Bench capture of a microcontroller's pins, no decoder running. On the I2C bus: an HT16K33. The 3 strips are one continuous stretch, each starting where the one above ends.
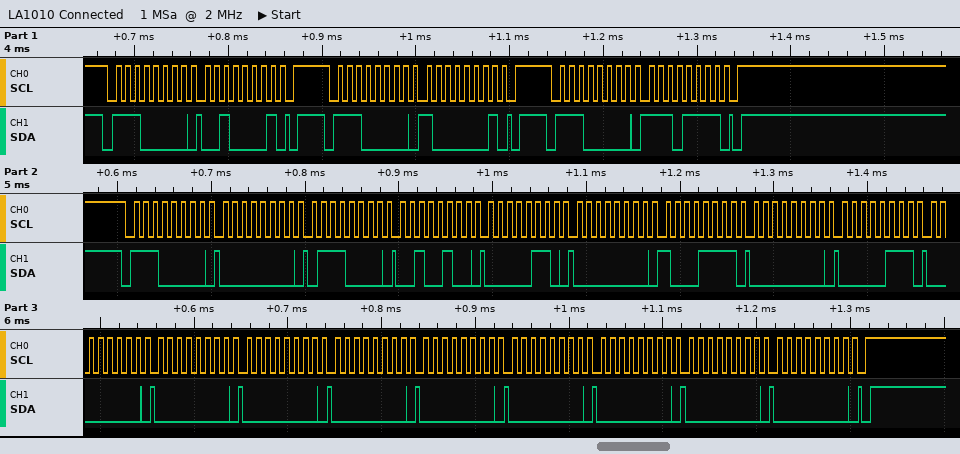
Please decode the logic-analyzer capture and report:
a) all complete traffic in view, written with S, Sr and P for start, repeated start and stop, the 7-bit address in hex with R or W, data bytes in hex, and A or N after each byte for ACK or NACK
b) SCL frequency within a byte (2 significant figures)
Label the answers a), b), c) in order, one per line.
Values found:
a) S 70W A 21 A P S 70W A 81 A P S 70W A EF A P S 70W A 00 A 70 A 24 A 06 A 00 A 8F A 00 A 07 A 00 A 00 A 00 A 00 A 00 A 00 A 00 A 00 A 00 A P
b) 100 kHz
